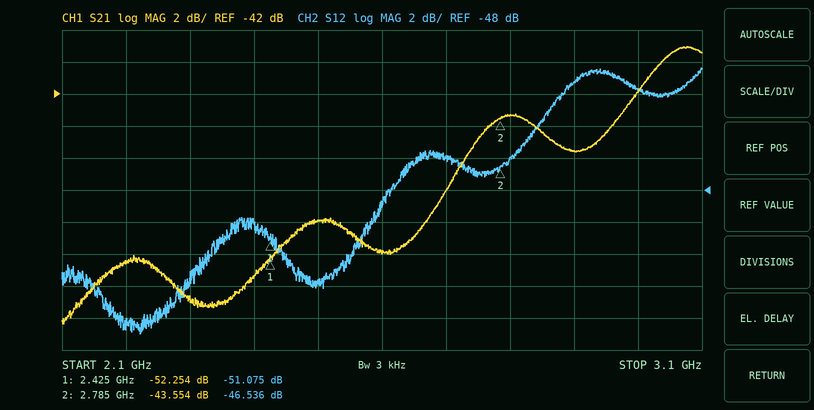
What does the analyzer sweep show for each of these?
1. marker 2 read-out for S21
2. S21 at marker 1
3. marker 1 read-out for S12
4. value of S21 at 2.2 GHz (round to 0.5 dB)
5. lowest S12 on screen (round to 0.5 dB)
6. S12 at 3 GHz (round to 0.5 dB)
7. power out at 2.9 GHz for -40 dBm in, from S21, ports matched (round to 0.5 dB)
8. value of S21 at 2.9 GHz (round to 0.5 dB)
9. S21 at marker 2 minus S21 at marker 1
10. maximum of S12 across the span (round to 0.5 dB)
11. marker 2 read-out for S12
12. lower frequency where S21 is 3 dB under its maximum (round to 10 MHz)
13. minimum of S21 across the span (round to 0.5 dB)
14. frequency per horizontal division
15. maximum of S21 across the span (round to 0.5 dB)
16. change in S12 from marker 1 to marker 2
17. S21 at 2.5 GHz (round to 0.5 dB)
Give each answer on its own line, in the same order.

-43.554 dB
-52.254 dB
-51.075 dB
-52.5 dB
-57.0 dB
-41.5 dB
-85.5 dBm
-45.5 dB
8.700 dB
-40.5 dB
-46.536 dB
3.00 GHz
-56.5 dB
100 MHz
-39.0 dB
4.539 dB
-50.0 dB
